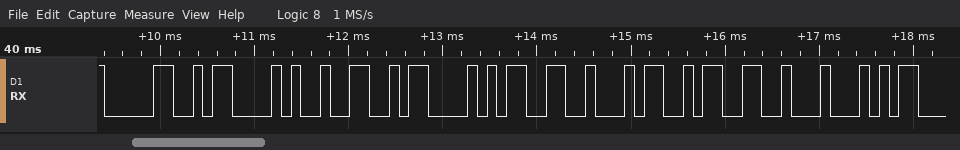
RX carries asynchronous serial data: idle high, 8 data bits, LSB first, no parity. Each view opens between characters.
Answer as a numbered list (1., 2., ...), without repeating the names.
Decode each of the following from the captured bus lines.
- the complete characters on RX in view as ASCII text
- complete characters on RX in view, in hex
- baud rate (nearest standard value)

1. "0C2C343D"
2. 30, 43, 32, 43, 33, 34, 33, 44
3. 9600 baud
